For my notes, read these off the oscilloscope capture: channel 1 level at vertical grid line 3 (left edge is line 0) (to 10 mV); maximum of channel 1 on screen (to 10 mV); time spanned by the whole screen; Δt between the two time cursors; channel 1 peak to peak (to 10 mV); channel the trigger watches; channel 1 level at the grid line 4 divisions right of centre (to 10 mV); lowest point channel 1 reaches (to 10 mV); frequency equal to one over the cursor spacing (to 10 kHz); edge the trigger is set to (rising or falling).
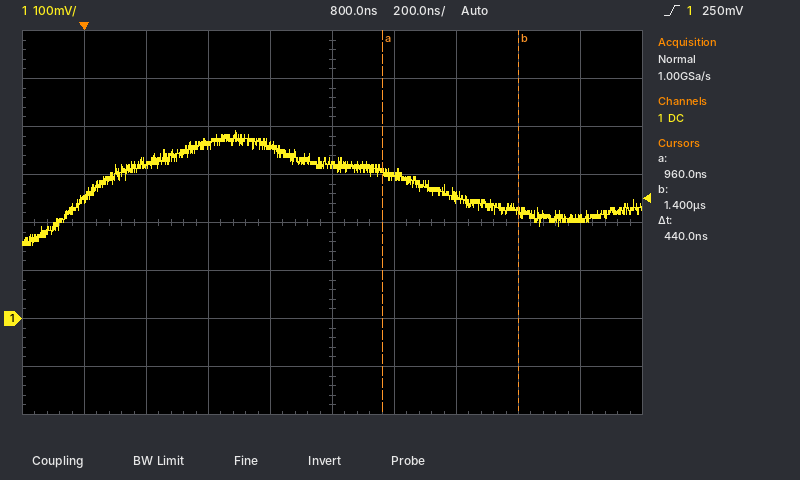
360 mV
390 mV
2 µs
440 ns
240 mV
channel 1
210 mV
150 mV
2.27 MHz
rising
